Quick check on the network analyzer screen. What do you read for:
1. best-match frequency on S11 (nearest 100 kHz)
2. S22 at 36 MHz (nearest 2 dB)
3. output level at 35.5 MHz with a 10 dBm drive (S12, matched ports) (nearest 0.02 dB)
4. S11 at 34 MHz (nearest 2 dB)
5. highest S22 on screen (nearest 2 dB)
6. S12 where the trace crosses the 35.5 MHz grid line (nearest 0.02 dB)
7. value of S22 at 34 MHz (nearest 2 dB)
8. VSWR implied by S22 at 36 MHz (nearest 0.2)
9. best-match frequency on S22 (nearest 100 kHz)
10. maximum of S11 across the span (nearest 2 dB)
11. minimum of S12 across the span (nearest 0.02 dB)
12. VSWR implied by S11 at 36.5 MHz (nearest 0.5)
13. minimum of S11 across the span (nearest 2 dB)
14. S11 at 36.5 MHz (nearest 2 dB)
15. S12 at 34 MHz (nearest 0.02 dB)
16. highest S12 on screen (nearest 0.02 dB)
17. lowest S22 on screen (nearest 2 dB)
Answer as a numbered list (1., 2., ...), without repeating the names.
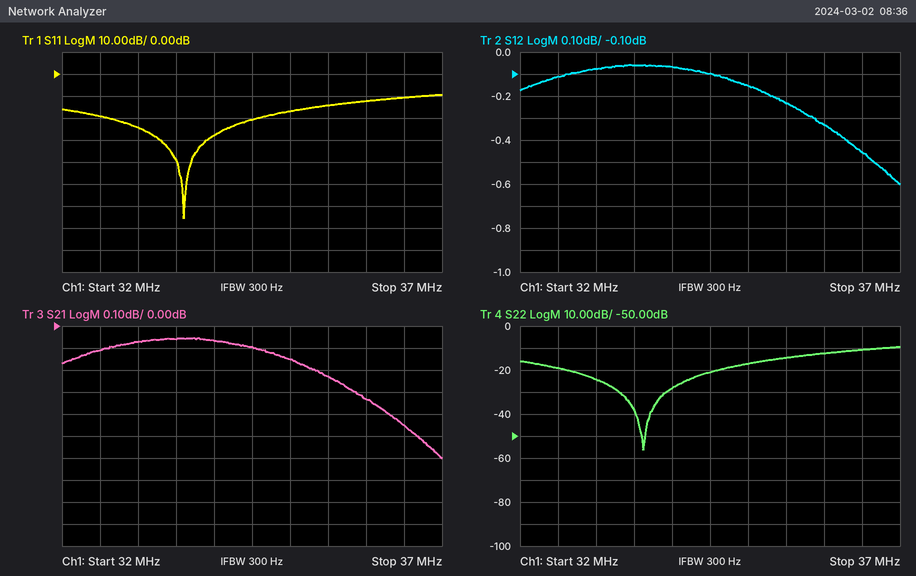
1. 33.6 MHz
2. -12 dB
3. 9.76 dBm
4. -28 dB
5. -10 dB
6. -0.24 dB
7. -28 dB
8. 1.6
9. 33.6 MHz
10. -10 dB
11. -0.60 dB
12. 2.0
13. -66 dB
14. -10 dB
15. -0.06 dB
16. -0.06 dB
17. -56 dB
